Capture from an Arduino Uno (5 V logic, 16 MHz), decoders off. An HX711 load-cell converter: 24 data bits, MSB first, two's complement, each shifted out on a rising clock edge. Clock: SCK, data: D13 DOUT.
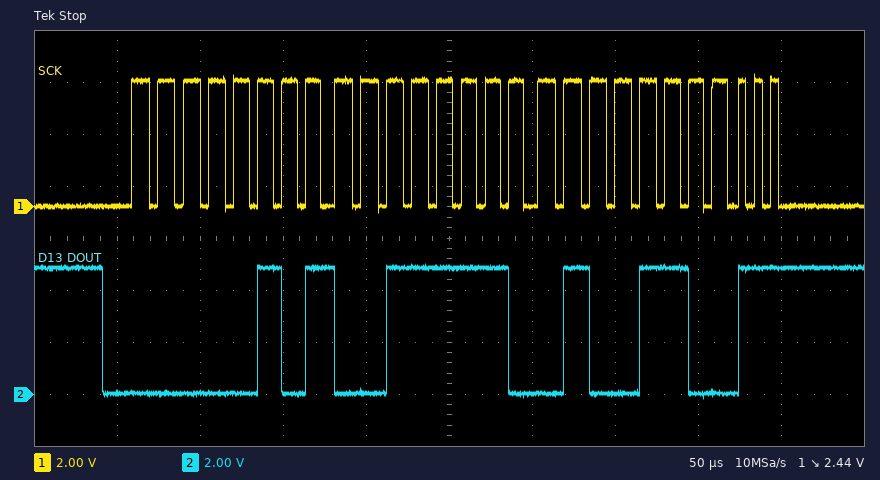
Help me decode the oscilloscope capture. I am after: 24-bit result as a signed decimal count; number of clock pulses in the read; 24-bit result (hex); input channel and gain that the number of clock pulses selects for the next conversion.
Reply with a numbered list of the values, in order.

1. 343628
2. 27
3. 0x053E4C
4. channel A, gain 64
